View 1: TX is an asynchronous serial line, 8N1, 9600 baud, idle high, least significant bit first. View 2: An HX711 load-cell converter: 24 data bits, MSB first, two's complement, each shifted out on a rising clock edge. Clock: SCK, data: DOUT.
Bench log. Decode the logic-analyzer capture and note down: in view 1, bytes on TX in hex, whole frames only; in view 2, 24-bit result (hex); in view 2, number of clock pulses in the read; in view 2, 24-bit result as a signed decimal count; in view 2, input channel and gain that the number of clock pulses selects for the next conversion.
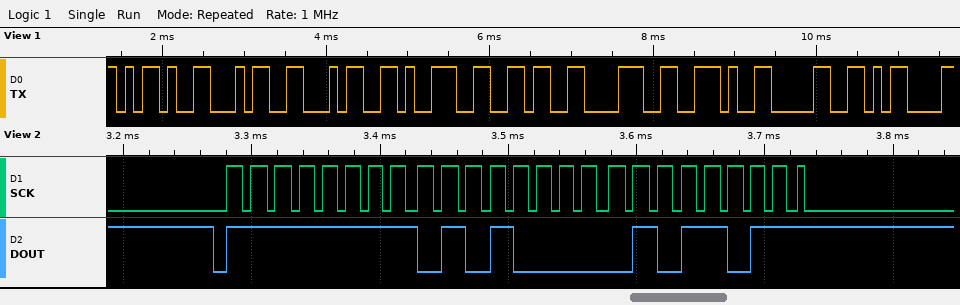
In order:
2D 34 34 39 36 38 2E 30 0D
0xFF505B
25
-44965
channel A, gain 128
